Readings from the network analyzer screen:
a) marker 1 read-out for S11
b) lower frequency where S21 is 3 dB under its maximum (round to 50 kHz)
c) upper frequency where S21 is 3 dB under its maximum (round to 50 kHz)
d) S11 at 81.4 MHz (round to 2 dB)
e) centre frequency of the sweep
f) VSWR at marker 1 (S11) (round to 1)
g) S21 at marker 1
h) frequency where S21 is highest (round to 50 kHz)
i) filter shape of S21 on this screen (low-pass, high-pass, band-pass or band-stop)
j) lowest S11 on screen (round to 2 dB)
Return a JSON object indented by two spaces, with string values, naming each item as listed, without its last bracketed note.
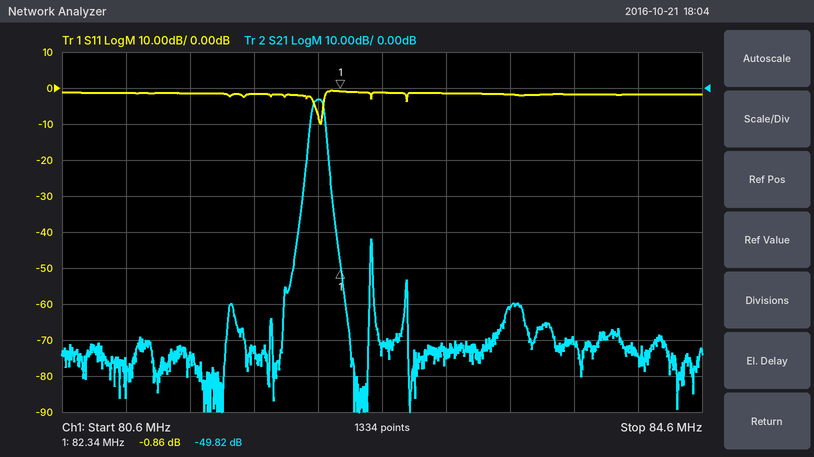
{
  "marker 1 read-out for S11": "-0.86 dB",
  "lower frequency where S21 is 3 dB under its maximum": "82.15 MHz",
  "upper frequency where S21 is 3 dB under its maximum": "82.25 MHz",
  "S11 at 81.4 MHz": "-2 dB",
  "centre frequency of the sweep": "82.6 MHz",
  "VSWR at marker 1 (S11)": "20",
  "S21 at marker 1": "-49.82 dB",
  "frequency where S21 is highest": "82.20 MHz",
  "filter shape of S21 on this screen": "band-pass",
  "lowest S11 on screen": "-10 dB"
}
